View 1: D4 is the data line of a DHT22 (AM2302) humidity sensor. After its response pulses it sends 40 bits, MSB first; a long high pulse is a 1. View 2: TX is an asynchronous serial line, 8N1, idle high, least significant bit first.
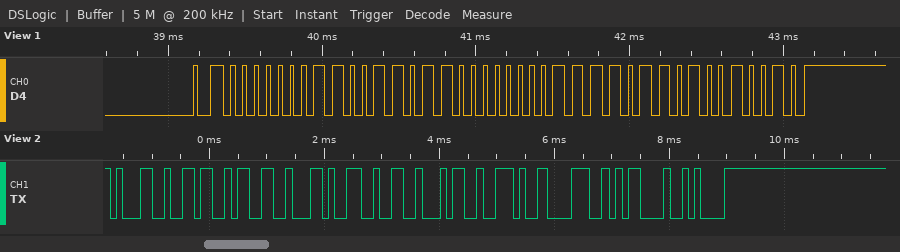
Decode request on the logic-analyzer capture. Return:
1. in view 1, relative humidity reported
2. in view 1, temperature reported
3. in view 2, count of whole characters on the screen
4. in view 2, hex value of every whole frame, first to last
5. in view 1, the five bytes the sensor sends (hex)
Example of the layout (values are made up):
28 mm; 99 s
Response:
41.1 %; 24.6 °C; 10; 31 36 33 2C 32 34 2E 38 0D 0A; 01 9B 00 F6 92
